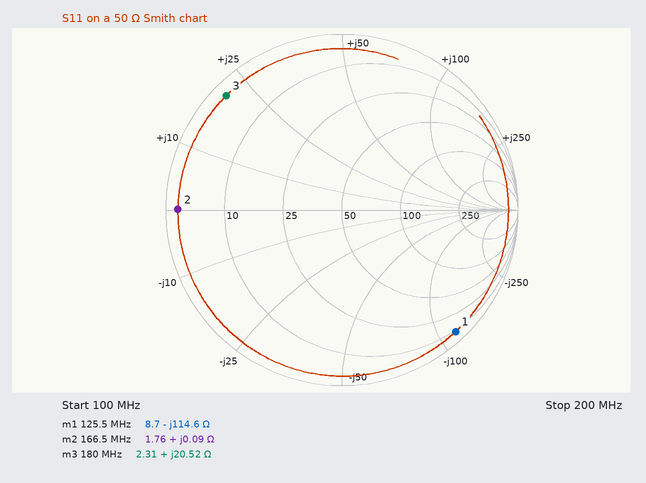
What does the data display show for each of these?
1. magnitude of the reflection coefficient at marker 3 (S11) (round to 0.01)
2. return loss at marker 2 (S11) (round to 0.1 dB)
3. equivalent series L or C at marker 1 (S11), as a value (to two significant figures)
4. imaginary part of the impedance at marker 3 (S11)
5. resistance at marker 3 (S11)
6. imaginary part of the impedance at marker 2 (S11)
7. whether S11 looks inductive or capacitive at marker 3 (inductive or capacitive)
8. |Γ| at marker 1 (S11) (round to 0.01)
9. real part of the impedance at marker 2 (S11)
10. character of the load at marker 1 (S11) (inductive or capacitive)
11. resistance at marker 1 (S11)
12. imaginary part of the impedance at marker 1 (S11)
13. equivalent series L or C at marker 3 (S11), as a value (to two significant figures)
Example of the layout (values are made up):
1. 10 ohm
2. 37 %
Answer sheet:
1. 0.92
2. 0.6 dB
3. 11 pF
4. +20.52 Ω
5. 2.31 Ω
6. +0.09 Ω
7. inductive
8. 0.95
9. 1.76 Ω
10. capacitive
11. 8.7 Ω
12. -114.6 Ω
13. 18 nH
